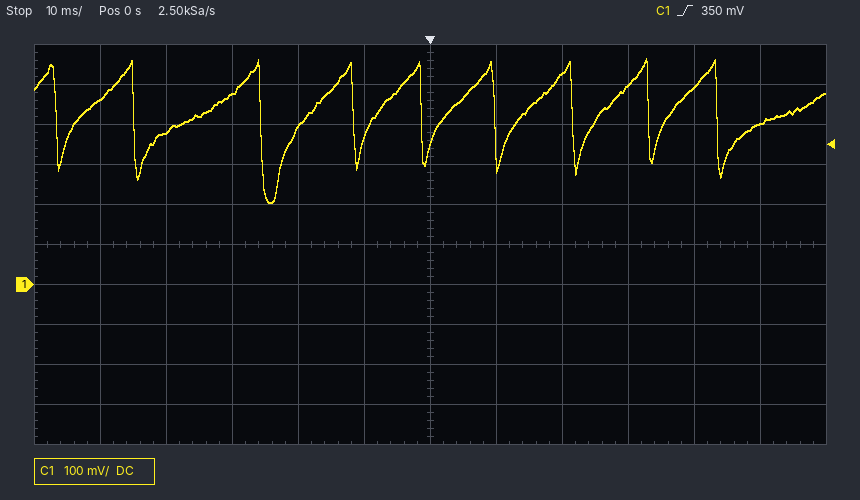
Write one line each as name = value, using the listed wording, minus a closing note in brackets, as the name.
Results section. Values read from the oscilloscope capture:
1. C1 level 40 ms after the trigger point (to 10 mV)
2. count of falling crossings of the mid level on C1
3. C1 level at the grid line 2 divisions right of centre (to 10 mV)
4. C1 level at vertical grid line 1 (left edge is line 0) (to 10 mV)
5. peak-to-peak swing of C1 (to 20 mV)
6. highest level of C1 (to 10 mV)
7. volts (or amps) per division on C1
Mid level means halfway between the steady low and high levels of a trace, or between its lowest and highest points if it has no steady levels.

C1 level 40 ms after the trigger point = 490 mV
count of falling crossings of the mid level on C1 = 9
C1 level at the grid line 2 divisions right of centre = 530 mV
C1 level at vertical grid line 1 (left edge is line 0) = 460 mV
peak-to-peak swing of C1 = 360 mV
highest level of C1 = 570 mV
volts (or amps) per division on C1 = 100 mV
